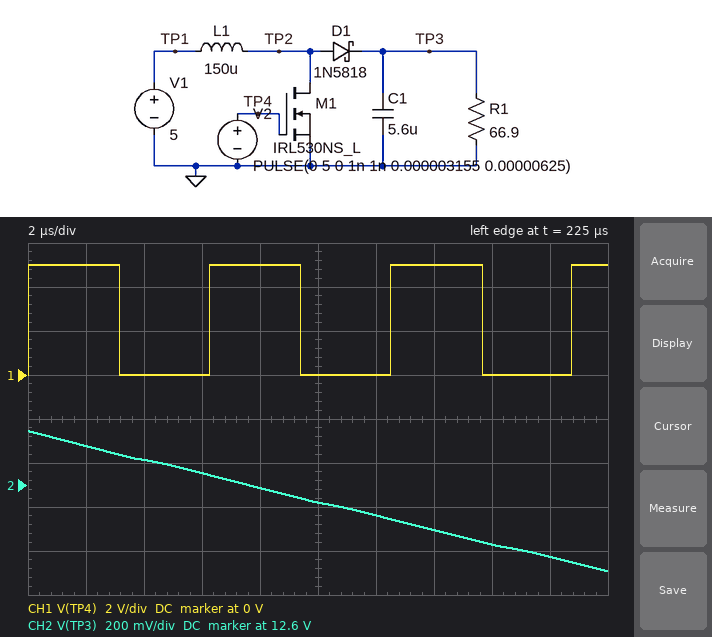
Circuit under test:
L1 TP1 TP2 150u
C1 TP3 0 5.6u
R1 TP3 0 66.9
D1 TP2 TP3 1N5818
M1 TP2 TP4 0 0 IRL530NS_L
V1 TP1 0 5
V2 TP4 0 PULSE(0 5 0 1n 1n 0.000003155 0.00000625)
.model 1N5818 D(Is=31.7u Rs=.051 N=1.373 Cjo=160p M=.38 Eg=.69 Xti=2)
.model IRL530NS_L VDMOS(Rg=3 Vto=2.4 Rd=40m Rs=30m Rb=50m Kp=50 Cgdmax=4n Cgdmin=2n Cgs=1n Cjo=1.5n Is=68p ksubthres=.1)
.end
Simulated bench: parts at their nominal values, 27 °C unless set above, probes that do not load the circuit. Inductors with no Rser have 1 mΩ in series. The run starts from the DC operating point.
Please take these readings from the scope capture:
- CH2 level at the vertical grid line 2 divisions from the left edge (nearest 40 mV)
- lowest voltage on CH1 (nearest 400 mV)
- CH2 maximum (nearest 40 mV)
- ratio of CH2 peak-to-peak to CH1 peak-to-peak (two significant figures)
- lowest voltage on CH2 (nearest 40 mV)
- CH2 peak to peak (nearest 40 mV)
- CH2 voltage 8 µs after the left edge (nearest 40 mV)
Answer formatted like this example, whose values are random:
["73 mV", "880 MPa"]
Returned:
["12.72 V", "0 V", "12.84 V", "0.13", "12.20 V", "640 mV", "12.60 V"]
